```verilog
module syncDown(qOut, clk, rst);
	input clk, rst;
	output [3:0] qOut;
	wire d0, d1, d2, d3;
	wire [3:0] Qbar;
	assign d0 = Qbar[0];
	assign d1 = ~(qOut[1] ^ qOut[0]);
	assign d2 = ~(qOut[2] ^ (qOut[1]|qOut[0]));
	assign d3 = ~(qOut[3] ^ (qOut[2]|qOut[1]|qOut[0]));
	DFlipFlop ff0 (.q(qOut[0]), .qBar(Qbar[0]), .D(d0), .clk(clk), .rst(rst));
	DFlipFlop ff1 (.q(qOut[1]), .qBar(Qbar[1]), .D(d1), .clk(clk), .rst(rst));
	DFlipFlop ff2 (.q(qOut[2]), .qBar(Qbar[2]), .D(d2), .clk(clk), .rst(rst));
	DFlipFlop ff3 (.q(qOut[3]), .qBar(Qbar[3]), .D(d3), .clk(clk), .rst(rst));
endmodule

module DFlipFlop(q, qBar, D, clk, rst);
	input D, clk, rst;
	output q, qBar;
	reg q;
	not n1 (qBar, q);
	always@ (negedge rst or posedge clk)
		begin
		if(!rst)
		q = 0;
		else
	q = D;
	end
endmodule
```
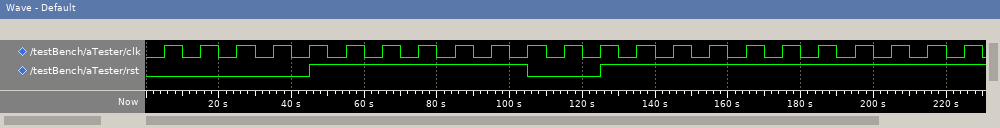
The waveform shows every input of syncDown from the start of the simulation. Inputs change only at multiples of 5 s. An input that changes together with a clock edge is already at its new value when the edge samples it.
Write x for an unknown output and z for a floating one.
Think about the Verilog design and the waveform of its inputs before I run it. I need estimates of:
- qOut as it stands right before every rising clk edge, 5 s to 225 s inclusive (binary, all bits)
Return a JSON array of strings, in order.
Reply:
["0000, 0000, 0000, 0000, 0000, 1111, 1110, 1101, 1100, 1011, 1010, 0000, 0000, 1111, 1110, 1101, 1100, 1011, 1010, 1001, 1000, 0111, 0110"]
